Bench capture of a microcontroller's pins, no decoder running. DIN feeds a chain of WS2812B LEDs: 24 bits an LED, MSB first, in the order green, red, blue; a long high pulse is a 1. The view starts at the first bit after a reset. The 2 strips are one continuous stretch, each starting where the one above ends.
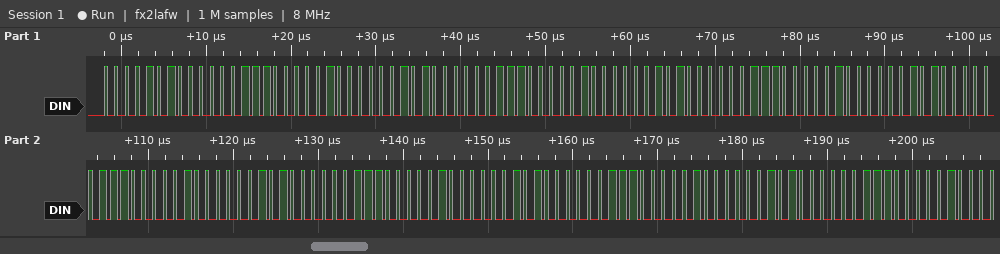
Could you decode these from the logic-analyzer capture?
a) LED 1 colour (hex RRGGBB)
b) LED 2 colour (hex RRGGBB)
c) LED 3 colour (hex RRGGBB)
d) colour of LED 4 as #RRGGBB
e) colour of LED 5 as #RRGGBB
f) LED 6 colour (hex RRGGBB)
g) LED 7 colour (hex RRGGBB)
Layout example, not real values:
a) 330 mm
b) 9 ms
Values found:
a) #070A04
b) #070A04
c) #070A04
d) #070A04
e) #070A04
f) #070A04
g) #070A04
